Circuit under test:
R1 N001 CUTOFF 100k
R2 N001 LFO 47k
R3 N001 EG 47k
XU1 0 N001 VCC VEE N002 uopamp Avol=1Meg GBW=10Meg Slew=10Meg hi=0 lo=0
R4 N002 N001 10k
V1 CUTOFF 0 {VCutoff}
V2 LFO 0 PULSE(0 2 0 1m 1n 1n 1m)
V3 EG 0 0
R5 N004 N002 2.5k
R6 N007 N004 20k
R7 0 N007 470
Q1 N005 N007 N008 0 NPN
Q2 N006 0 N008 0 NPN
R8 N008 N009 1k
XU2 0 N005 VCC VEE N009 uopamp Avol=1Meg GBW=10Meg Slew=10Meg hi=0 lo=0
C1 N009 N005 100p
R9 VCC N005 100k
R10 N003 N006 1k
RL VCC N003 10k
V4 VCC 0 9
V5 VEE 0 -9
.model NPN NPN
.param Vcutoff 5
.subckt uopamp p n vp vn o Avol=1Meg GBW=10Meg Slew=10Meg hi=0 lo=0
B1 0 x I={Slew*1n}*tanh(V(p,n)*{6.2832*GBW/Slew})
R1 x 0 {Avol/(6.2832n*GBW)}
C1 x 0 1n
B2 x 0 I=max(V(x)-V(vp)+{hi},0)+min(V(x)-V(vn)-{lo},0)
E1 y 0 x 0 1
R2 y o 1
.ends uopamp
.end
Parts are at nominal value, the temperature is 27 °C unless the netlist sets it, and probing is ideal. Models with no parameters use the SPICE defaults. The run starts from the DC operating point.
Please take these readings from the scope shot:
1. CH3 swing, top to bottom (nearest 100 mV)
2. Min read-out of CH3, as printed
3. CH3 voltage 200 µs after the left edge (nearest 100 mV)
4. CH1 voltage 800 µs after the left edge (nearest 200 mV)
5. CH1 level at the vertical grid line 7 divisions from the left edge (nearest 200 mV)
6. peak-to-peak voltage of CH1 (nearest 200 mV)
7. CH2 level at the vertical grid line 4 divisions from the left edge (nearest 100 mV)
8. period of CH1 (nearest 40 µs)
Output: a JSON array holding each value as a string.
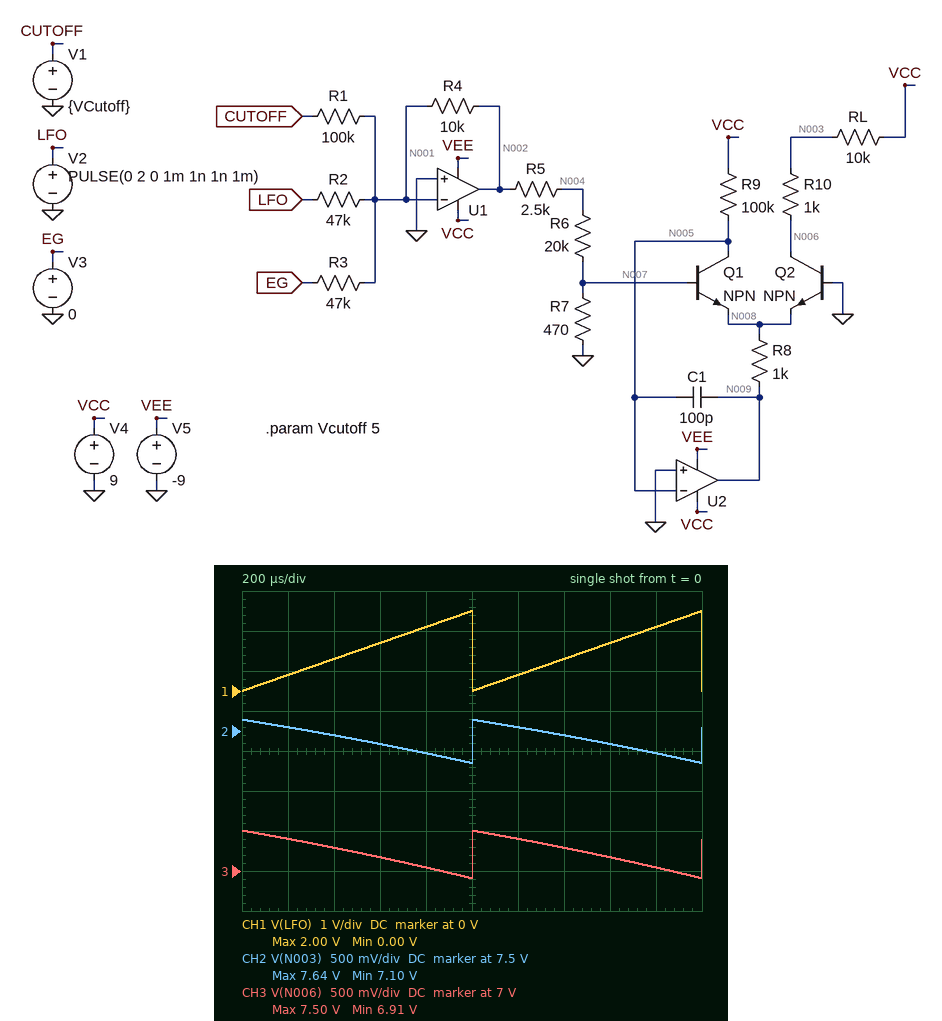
["600 mV", "6.91 V", "7.4 V", "1.6 V", "800 mV", "2.0 V", "7.2 V", "1.00 ms"]
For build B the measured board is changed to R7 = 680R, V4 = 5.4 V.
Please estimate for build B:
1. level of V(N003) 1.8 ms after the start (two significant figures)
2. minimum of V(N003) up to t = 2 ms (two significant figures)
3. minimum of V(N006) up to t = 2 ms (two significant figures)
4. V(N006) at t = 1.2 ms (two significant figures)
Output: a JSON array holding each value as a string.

["4.0 V", "3.8 V", "3.7 V", "4.2 V"]
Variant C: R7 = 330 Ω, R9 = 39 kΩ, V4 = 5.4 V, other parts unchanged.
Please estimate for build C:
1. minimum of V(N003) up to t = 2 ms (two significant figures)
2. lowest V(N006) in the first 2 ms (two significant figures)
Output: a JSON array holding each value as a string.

["3.0 V", "2.8 V"]
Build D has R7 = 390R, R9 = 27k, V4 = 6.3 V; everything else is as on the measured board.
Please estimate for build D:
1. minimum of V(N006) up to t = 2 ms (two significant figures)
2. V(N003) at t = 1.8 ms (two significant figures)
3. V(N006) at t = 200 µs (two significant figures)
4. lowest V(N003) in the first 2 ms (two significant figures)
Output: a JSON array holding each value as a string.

["1.4 V", "2.1 V", "2.4 V", "1.9 V"]
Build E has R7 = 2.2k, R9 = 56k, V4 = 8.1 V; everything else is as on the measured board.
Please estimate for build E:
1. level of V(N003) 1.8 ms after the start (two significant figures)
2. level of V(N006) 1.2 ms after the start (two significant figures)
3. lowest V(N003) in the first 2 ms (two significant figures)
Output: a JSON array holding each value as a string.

["31 mV", "-730 mV", "22 mV"]
